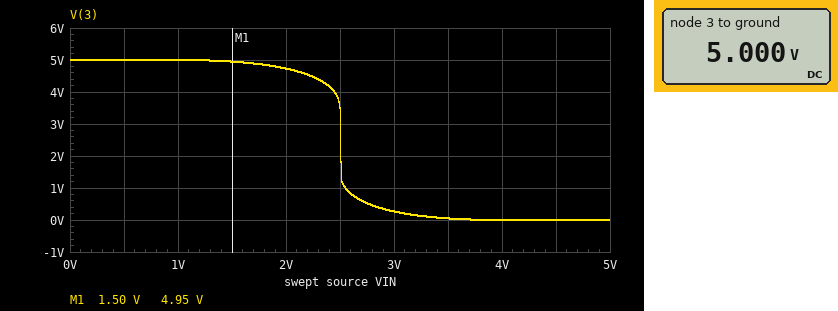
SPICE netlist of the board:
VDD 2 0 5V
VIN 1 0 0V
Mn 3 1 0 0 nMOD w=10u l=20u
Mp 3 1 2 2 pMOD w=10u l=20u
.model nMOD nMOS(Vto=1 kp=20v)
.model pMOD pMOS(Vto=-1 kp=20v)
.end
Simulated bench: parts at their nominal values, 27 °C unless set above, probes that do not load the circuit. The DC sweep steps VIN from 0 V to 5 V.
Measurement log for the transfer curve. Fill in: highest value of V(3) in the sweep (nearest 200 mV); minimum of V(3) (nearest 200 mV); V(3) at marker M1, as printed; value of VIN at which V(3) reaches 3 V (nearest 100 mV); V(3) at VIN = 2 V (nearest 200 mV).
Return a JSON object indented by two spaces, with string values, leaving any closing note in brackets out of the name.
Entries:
{
  "highest value of V(3) in the sweep": "5.0 V",
  "minimum of V(3)": "0 V",
  "V(3) at marker M1, as printed": "4.95 V",
  "value of VIN at which V(3) reaches 3 V": "2.5 V",
  "V(3) at VIN = 2 V": "4.8 V"
}
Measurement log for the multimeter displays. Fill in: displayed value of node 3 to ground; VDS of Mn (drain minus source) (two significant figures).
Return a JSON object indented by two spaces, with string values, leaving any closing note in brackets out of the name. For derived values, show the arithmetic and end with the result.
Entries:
{
  "displayed value of node 3 to ground": "5.000 V",
  "VDS of Mn (drain minus source)": "5 V = 5.0 V"
}
